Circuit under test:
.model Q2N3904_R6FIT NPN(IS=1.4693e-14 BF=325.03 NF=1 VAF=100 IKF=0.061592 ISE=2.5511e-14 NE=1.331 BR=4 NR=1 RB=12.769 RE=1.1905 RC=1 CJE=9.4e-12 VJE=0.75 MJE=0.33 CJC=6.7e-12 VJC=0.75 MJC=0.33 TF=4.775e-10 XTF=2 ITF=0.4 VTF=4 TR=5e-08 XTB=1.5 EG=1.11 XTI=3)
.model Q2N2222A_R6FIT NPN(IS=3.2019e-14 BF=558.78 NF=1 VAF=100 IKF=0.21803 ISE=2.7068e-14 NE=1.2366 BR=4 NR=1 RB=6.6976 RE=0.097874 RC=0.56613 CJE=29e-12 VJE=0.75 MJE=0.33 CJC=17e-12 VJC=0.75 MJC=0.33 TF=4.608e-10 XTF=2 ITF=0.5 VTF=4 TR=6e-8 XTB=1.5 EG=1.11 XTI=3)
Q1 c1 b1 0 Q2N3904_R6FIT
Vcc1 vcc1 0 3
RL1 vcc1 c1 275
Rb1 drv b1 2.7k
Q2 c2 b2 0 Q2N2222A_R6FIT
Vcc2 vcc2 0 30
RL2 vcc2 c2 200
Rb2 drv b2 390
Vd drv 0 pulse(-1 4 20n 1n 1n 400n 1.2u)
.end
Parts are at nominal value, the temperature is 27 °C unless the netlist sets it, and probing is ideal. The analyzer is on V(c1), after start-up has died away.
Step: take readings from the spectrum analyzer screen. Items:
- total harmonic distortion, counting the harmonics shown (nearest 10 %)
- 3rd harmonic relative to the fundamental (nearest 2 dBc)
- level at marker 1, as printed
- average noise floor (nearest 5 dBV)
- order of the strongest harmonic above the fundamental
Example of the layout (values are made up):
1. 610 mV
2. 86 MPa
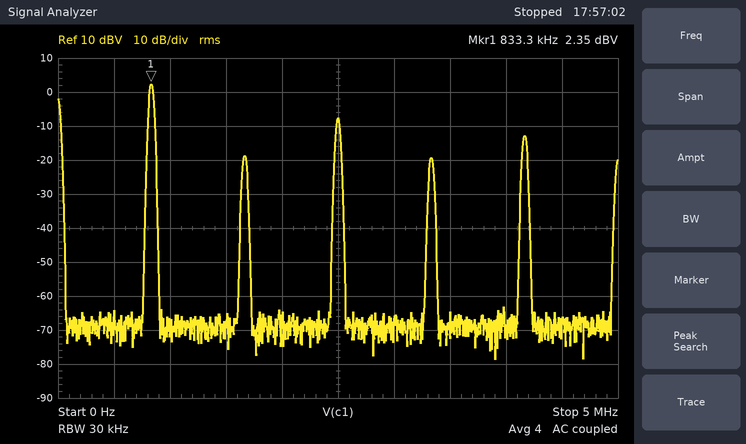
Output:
1. 40 %
2. -10 dBc
3. 2.35 dBV
4. -70 dBV
5. 3
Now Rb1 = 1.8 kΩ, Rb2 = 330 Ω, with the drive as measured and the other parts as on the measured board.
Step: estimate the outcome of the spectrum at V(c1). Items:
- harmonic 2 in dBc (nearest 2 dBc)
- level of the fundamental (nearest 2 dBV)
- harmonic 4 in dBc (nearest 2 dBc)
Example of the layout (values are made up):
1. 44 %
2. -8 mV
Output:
1. -24 dBc
2. 2 dBV
3. -24 dBc
